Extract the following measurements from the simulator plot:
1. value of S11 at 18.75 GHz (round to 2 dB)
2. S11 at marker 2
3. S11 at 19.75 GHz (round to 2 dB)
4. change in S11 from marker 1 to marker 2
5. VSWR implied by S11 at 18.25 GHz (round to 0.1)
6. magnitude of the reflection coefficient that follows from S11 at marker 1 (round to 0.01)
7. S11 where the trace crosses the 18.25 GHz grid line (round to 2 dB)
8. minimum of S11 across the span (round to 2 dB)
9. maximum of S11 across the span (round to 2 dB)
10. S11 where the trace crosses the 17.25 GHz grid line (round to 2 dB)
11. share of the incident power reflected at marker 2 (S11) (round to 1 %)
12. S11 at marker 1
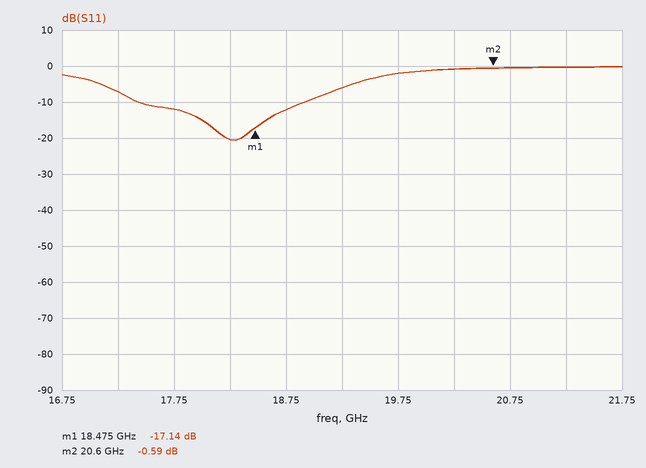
-12 dB
-0.59 dB
-2 dB
16.55 dB
1.2
0.14
-20 dB
-20 dB
0 dB
-8 dB
87 %
-17.14 dB
